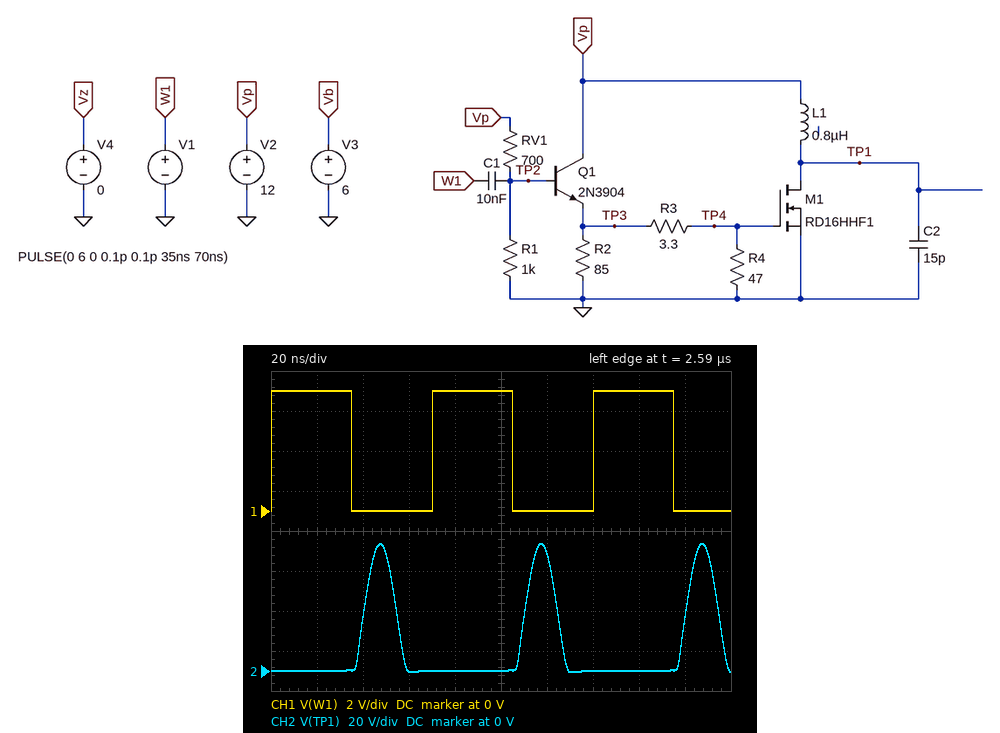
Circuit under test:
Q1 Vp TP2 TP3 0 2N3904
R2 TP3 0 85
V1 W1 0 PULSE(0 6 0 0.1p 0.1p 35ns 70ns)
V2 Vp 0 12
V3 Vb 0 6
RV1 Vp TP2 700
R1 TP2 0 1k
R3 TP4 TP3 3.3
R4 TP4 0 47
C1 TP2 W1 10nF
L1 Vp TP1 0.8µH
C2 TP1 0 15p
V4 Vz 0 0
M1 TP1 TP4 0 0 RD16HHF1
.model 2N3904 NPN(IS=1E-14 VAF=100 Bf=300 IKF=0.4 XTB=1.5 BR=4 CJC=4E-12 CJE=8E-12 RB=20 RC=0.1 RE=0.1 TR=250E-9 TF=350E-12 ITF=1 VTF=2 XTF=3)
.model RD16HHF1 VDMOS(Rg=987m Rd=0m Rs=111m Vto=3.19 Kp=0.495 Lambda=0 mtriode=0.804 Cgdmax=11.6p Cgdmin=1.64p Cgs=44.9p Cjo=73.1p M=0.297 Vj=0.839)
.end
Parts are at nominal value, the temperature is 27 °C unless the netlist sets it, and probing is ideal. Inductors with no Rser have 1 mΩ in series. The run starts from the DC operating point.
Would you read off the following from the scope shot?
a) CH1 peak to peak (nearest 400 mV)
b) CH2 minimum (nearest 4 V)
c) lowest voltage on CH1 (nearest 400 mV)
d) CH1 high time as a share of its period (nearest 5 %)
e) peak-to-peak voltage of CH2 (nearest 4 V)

6.0 V
0 V
0 V
50 %
64 V
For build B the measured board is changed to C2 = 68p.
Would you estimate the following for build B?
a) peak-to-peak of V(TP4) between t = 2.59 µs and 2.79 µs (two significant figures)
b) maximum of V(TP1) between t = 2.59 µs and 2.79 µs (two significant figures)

6.3 V
38 V
